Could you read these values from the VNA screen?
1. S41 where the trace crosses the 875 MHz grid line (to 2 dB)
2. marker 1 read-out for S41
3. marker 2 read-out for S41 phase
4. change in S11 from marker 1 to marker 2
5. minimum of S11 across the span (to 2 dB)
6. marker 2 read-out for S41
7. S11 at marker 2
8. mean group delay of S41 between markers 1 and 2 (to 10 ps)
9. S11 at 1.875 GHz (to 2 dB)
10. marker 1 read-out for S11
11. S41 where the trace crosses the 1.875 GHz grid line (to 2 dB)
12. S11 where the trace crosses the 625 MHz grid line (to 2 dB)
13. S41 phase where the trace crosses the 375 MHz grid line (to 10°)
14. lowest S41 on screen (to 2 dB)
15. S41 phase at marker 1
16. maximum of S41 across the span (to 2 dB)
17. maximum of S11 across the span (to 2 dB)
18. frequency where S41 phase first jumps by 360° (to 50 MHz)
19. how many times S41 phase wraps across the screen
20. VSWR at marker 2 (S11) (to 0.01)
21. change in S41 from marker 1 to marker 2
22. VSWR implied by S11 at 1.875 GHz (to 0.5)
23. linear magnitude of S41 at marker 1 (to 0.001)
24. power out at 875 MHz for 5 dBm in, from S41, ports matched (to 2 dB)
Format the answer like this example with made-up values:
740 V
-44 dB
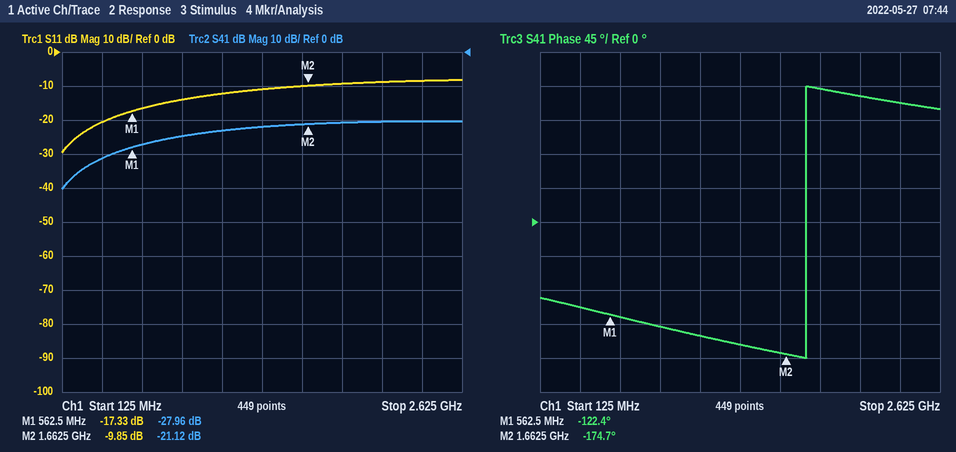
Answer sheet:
-24 dB
-27.96 dB
-174.7°
7.48 dB
-30 dB
-21.12 dB
-9.85 dB
130 ps
-10 dB
-17.33 dB
-20 dB
-16 dB
-110°
-40 dB
-122.4°
-20 dB
-8 dB
1.80 GHz
1
1.95
6.84 dB
2.0
0.040
-20 dBm
